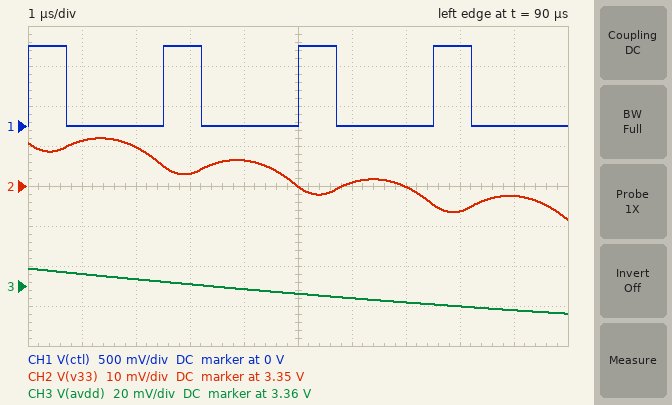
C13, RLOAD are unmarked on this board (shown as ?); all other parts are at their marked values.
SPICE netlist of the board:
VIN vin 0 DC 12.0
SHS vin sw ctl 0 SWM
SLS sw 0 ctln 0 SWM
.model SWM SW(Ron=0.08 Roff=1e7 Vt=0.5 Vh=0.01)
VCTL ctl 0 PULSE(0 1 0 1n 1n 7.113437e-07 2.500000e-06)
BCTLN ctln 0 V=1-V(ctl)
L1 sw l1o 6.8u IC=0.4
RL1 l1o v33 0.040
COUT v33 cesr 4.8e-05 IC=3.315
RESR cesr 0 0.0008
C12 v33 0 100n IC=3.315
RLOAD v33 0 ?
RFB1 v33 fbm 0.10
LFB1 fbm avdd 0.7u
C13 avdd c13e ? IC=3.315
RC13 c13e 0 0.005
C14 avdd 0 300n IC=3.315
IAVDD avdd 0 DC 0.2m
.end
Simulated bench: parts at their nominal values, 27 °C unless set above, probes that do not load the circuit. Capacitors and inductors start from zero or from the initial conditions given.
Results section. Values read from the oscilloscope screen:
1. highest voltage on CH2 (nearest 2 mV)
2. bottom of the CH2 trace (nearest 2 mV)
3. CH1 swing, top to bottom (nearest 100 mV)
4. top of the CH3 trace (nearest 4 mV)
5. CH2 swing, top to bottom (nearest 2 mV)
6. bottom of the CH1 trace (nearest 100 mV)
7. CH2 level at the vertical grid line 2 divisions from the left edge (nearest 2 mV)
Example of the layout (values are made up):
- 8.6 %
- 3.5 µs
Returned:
- 3.362 V
- 3.342 V
- 1.0 V
- 3.368 V
- 20 mV
- 0 V
- 3.360 V
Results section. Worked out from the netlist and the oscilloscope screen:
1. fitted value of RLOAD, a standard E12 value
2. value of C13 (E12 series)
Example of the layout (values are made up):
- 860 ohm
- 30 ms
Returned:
- 12 Ω
- 27 µF
